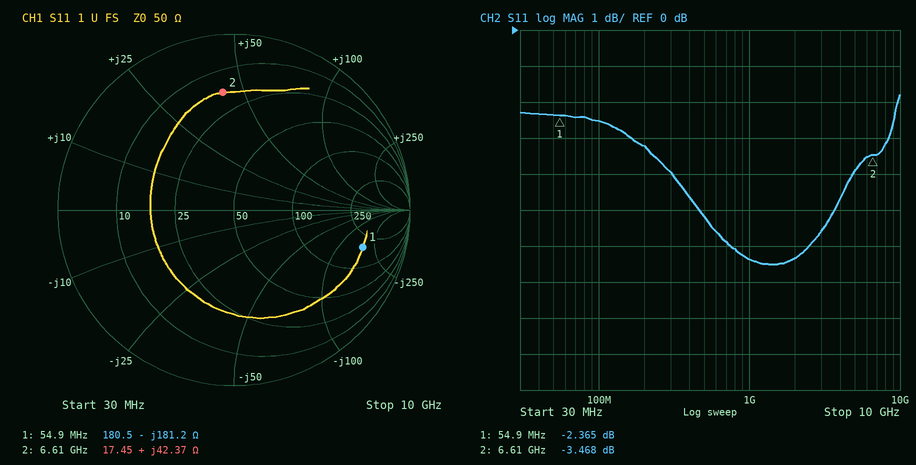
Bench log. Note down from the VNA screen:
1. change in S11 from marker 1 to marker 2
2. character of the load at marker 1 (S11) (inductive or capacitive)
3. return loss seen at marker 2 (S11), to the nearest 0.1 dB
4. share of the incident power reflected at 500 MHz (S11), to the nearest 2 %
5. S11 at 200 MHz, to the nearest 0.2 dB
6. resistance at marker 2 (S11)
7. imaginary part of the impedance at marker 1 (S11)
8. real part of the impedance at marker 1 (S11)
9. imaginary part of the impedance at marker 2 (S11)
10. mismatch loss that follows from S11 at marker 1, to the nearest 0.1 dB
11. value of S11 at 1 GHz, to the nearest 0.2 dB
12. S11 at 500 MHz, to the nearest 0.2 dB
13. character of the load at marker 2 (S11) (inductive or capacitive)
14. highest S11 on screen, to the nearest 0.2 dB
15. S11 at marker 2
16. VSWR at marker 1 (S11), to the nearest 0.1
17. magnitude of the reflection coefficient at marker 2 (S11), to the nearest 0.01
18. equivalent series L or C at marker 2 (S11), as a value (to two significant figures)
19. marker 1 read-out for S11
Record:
-1.103 dB
capacitive
3.5 dB
30 %
-3.2 dB
17.45 Ω
-181.2 Ω
180.5 Ω
+42.37 Ω
3.8 dB
-6.4 dB
-5.2 dB
inductive
-1.8 dB
-3.468 dB
7.4
0.67
1.0 nH
-2.365 dB
